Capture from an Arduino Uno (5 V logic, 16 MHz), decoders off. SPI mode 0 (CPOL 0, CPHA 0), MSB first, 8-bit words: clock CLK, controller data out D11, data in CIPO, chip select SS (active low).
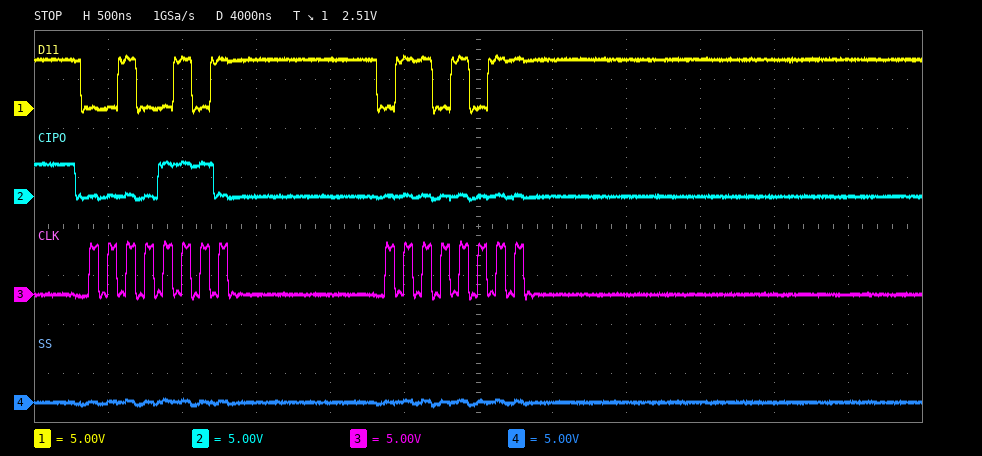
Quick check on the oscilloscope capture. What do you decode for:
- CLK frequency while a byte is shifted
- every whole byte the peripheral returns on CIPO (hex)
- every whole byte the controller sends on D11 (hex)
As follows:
8 MHz
0E 00
25 6B
